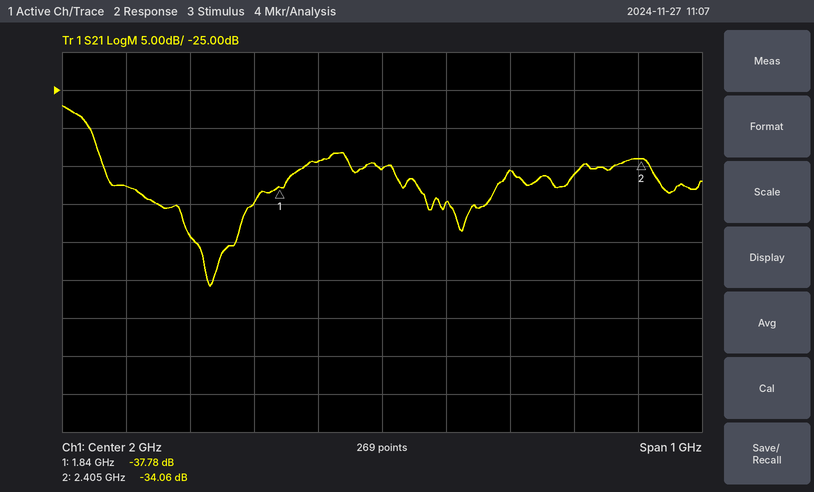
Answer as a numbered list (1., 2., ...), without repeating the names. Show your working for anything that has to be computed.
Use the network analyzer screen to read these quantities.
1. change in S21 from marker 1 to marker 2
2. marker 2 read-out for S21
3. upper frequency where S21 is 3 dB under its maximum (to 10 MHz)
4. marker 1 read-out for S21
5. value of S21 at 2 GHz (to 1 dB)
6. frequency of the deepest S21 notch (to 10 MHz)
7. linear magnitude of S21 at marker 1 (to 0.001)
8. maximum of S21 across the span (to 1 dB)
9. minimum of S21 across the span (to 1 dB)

1. -34.06 − (-37.78) = 3.72 dB
2. -34.06 dB
3. 1.54 GHz
4. -37.78 dB
5. -35 dB
6. 1.73 GHz
7. 10^(-37.78/20) ≈ 0.013
8. -27 dB
9. -51 dB
